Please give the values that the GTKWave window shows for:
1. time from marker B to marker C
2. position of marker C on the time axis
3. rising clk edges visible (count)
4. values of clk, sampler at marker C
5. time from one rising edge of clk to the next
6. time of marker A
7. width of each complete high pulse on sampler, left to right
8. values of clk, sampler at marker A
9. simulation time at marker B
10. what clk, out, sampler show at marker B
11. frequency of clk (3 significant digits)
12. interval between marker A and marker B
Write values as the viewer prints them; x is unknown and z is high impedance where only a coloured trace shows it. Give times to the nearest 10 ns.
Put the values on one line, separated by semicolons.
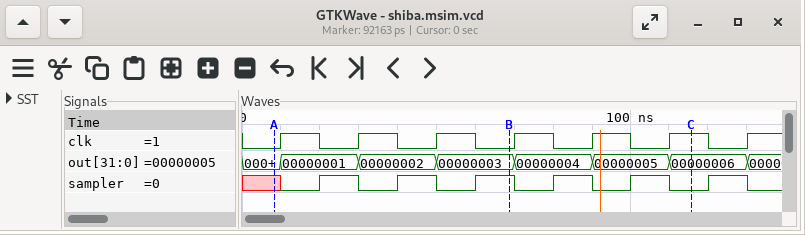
50 ns; 120 ns; 7; clk=1, sampler=0; 20 ns; 10 ns; 10 ns, 10 ns, 10 ns, 10 ns, 10 ns, 10 ns; clk=0, sampler=x; 70 ns; clk=0, out=00000003, sampler=1; 50.0 MHz; 60 ns
